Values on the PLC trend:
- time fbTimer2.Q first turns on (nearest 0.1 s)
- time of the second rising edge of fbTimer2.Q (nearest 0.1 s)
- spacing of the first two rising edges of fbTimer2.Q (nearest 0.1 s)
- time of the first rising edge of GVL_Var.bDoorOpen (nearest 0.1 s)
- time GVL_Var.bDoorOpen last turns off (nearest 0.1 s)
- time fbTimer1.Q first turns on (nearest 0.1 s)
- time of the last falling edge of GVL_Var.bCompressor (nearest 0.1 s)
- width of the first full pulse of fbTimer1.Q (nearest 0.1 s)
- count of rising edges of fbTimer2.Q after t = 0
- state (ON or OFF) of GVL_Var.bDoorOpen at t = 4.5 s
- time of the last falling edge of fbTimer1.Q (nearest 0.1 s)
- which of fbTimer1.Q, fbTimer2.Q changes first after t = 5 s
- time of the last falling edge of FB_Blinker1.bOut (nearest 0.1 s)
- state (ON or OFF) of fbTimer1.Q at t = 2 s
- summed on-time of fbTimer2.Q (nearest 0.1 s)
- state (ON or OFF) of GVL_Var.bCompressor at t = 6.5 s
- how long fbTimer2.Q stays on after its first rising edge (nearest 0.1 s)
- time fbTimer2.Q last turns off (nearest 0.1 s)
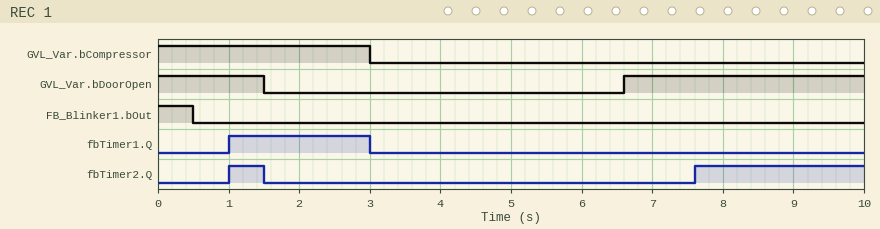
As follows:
1.0 s
7.6 s
6.6 s
6.6 s
1.5 s
1.0 s
3.0 s
2.0 s
2
OFF
3.0 s
fbTimer2.Q
0.5 s
ON
2.9 s
OFF
0.5 s
1.5 s
